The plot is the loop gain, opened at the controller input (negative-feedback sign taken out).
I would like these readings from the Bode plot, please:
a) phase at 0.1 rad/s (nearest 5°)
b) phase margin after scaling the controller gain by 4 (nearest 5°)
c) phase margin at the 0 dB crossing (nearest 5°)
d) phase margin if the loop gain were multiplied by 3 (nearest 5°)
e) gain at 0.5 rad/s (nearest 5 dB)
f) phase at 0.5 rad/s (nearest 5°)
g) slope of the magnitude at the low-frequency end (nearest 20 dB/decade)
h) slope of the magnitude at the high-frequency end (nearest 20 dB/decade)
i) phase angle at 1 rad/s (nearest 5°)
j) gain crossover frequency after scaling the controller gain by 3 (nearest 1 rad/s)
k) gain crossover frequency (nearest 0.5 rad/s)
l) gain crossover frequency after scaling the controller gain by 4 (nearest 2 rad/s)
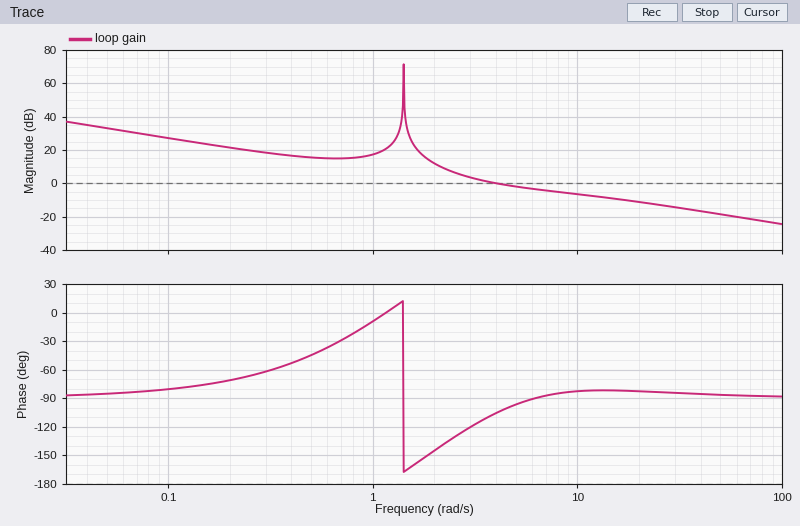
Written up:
-80°
95°
75°
100°
15 dB
-45°
-20 dB/decade
-20 dB/decade
-10°
16 rad/s
4.0 rad/s
22 rad/s
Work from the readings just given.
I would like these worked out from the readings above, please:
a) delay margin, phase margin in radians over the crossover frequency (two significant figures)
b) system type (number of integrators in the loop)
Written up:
0.33 s
1
